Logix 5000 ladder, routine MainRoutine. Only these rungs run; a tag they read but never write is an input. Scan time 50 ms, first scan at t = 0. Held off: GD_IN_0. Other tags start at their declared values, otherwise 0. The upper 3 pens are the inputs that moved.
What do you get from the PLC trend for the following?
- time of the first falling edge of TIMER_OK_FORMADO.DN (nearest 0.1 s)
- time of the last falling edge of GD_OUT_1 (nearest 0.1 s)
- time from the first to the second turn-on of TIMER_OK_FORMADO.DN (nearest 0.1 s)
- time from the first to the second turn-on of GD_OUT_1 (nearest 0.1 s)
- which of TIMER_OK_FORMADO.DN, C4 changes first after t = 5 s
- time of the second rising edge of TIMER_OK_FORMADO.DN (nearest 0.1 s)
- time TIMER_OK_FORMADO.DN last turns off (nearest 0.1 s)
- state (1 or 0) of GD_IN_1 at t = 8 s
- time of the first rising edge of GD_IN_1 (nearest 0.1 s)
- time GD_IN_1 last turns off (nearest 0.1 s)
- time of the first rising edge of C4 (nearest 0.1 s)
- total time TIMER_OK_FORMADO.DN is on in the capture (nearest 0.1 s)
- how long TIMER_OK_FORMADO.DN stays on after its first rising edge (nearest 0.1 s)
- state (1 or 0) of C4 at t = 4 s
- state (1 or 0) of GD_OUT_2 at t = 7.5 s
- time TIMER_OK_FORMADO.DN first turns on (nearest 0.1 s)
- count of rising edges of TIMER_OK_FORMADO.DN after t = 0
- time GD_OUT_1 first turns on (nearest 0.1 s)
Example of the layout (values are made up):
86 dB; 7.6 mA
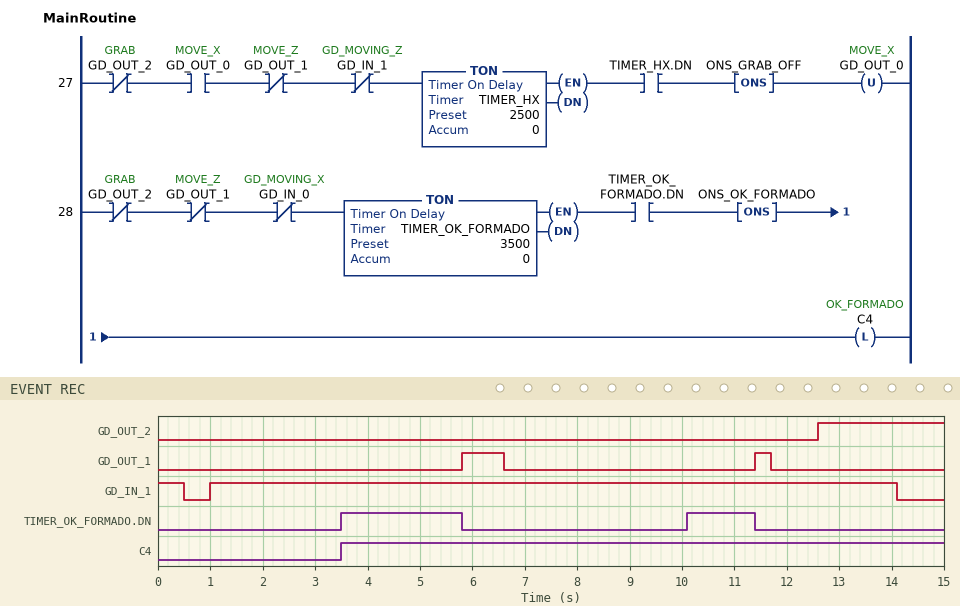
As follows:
5.8 s; 11.7 s; 6.6 s; 5.6 s; TIMER_OK_FORMADO.DN; 10.1 s; 11.4 s; 1; 1.0 s; 14.1 s; 3.5 s; 3.6 s; 2.3 s; 1; 0; 3.5 s; 2; 5.8 s
